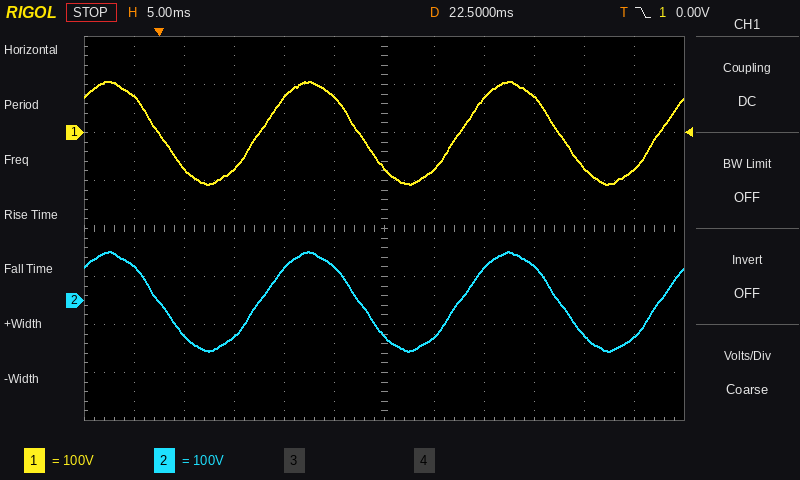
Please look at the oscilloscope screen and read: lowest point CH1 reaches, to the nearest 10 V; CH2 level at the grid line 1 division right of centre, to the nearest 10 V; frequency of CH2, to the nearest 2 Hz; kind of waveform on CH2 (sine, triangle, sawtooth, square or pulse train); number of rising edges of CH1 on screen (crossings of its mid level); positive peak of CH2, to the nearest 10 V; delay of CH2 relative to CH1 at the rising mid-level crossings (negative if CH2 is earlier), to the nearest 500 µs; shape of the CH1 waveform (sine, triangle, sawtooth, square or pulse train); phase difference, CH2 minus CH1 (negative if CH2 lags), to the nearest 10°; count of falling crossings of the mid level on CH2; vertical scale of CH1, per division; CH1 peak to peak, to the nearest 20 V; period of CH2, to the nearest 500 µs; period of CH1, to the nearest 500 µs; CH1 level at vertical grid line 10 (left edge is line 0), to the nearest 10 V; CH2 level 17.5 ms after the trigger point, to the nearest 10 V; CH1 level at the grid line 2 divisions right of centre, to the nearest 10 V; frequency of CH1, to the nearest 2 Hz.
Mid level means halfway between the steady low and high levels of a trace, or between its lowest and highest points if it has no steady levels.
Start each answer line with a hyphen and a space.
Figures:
- -110 V
- -80 V
- 50 Hz
- sine
- 3
- 100 V
- 0.0 ms
- sine
- 0°
- 3
- 100 V
- 220 V
- 20.0 ms
- 20.0 ms
- -70 V
- 70 V
- 70 V
- 50 Hz
